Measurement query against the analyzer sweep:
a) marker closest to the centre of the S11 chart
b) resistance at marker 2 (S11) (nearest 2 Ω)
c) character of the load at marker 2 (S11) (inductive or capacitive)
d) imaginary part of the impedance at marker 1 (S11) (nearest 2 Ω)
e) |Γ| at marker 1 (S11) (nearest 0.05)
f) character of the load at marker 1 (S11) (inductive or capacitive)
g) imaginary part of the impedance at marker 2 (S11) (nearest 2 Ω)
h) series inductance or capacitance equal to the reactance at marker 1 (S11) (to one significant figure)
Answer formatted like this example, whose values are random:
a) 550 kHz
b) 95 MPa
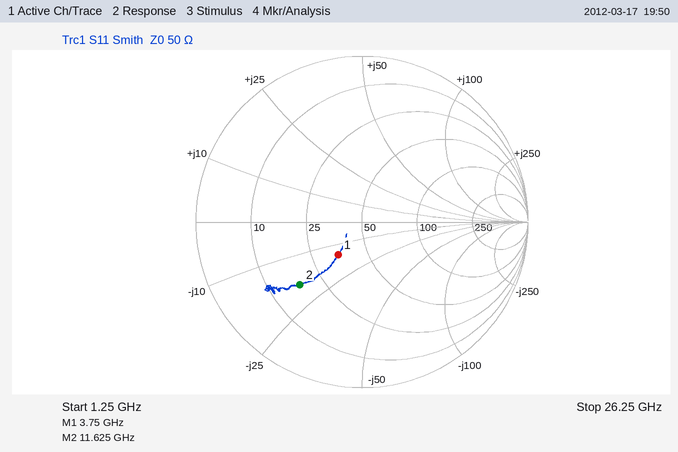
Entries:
a) marker 1
b) 18 Ω
c) capacitive
d) -14 Ω
e) 0.25
f) capacitive
g) -18 Ω
h) 3 pF
